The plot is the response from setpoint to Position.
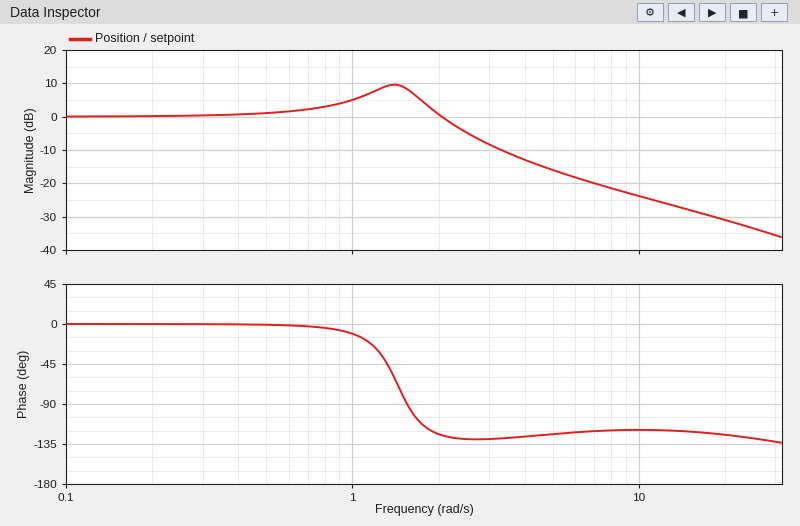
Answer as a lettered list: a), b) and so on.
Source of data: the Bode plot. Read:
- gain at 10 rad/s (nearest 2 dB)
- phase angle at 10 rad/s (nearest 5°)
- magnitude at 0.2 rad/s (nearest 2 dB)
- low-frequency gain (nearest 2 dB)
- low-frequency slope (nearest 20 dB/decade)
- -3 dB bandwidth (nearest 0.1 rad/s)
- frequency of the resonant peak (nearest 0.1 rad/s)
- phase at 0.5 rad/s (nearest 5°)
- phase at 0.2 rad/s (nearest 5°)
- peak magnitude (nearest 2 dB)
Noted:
a) -24 dB
b) -120°
c) 0 dB
d) 0 dB
e) 0 dB/decade
f) 2.3 rad/s
g) 1.4 rad/s
h) 0°
i) 0°
j) 10 dB
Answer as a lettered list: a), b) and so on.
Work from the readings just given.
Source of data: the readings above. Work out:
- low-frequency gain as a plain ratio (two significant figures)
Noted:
a) 1.0
